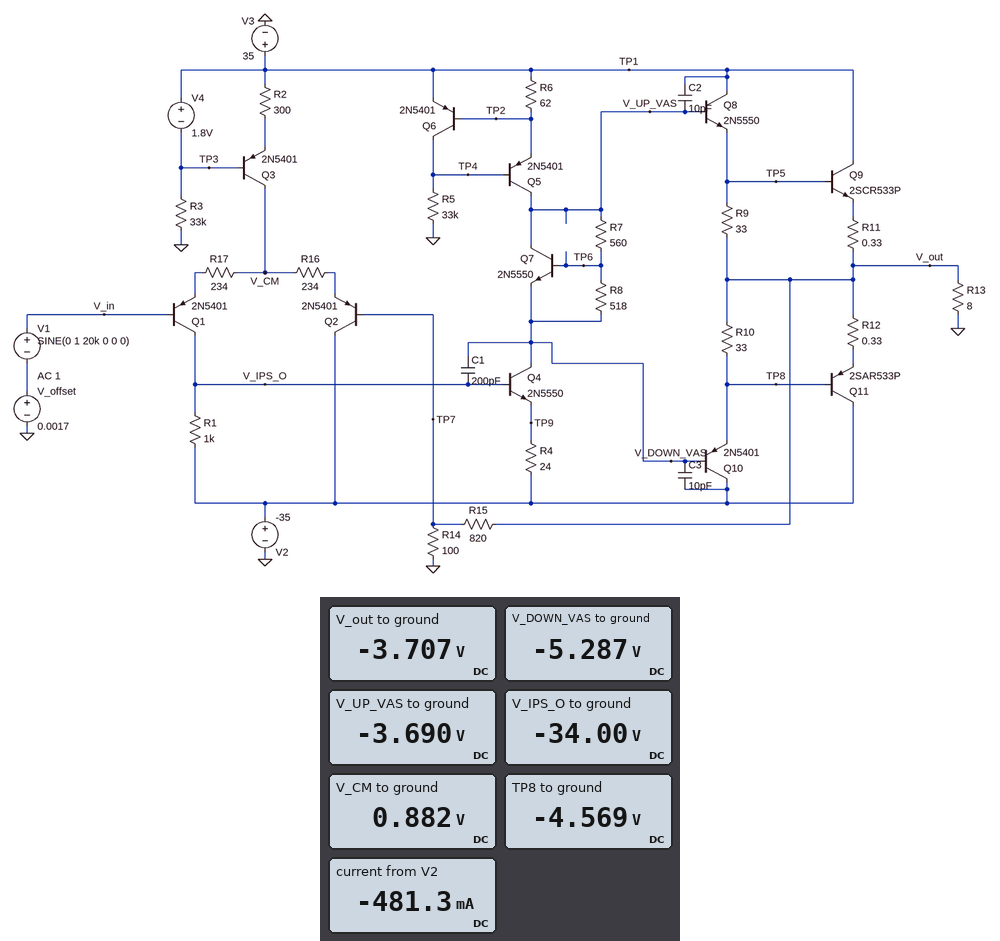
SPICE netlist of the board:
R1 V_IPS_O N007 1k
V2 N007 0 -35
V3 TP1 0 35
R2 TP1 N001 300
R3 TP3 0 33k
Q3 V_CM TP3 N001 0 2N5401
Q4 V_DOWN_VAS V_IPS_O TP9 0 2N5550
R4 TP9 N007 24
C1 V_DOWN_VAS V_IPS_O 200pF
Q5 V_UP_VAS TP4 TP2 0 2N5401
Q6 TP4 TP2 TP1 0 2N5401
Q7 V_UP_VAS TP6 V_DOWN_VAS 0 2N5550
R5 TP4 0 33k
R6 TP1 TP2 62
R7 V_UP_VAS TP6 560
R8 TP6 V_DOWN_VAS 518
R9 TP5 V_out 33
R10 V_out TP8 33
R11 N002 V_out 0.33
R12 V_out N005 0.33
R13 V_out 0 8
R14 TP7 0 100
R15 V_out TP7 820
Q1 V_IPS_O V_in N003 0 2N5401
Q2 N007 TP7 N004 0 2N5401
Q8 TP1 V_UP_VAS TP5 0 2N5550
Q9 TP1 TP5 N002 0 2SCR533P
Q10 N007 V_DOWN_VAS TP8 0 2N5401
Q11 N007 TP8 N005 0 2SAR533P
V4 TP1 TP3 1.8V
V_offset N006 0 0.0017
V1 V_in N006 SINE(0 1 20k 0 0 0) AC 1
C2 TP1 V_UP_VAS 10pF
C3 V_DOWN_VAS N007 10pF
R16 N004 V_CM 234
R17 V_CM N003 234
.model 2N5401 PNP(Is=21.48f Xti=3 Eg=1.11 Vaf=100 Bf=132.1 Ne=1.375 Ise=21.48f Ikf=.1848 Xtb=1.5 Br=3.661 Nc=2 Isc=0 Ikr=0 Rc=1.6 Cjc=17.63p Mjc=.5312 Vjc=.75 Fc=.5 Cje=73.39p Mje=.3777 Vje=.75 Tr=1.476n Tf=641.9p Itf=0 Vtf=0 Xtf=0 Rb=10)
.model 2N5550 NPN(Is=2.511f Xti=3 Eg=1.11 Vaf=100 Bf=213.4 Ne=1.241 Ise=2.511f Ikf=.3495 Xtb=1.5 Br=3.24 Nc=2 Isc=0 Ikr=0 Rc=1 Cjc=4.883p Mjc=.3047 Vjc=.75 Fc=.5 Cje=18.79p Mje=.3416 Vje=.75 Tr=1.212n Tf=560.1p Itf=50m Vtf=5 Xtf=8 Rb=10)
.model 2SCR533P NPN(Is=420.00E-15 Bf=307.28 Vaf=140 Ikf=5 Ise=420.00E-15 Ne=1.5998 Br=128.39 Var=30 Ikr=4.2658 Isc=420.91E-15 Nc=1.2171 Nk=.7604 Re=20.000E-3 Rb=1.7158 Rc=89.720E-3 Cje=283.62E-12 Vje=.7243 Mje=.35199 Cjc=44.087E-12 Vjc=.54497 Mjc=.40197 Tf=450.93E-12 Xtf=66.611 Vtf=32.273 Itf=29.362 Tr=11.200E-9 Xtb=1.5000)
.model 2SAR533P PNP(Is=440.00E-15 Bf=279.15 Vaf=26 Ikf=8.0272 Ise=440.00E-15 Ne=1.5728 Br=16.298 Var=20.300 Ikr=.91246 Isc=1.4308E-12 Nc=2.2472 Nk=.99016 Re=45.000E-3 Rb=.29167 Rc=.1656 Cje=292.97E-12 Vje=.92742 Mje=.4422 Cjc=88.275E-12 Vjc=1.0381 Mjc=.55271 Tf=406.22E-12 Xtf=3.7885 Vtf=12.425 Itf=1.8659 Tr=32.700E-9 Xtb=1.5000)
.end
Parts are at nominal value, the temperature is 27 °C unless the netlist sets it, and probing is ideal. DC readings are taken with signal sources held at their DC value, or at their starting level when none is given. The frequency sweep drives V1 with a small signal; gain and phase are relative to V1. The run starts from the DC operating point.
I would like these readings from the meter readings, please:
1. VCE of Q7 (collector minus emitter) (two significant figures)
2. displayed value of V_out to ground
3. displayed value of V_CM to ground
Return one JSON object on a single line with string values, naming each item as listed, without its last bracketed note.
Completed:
{"VCE of Q7 (collector minus emitter)": "1.6 V", "displayed value of V_out to ground": "-3.707 V", "displayed value of V_CM to ground": "0.882 V"}
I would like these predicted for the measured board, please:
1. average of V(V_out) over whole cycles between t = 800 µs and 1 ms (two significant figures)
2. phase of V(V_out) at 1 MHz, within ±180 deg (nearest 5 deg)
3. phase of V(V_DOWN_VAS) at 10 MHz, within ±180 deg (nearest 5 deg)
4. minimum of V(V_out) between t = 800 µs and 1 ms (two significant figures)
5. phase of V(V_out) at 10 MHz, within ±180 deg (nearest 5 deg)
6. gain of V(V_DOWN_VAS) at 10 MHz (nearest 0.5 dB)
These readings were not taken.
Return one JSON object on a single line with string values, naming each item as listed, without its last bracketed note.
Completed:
{"average of V(V_out) over whole cycles between t = 800 µs and 1 ms": "-3.7 V", "phase of V(V_out) at 1 MHz, within ±180 deg": "-85 deg", "phase of V(V_DOWN_VAS) at 10 MHz, within ±180 deg": "-130 deg", "minimum of V(V_out) between t = 800 µs and 1 ms": "-13 V", "phase of V(V_out) at 10 MHz, within ±180 deg": "-130 deg", "gain of V(V_DOWN_VAS) at 10 MHz": "-16.0 dB"}
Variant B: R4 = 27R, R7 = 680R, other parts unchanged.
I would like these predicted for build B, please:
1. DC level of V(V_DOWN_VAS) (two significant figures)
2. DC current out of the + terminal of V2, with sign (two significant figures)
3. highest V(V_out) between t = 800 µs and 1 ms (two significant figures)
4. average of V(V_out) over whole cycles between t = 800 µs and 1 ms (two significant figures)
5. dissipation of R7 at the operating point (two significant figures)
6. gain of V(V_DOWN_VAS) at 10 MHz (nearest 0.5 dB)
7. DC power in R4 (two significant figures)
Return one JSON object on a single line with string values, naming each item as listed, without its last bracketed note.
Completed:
{"DC level of V(V_DOWN_VAS)": "-5.1 V", "DC current out of the + terminal of V2, with sign": "-460 mA", "highest V(V_out) between t = 800 µs and 1 ms": "5.5 V", "average of V(V_out) over whole cycles between t = 800 µs and 1 ms": "-3.6 V", "dissipation of R7 at the operating point": "1.6 mW", "gain of V(V_DOWN_VAS) at 10 MHz": "-15.5 dB", "DC power in R4": "2.9 mW"}
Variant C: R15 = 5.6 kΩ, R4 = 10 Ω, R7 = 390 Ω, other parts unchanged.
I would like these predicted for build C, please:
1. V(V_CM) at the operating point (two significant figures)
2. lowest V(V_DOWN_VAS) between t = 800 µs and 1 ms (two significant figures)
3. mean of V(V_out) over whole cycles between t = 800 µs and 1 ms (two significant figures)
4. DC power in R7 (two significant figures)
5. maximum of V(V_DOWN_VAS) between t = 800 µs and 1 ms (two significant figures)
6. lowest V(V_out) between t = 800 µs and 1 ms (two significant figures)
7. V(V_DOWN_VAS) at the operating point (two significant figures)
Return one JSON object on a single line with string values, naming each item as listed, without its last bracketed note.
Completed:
{"V(V_CM) at the operating point": "850 mV", "lowest V(V_DOWN_VAS) between t = 800 µs and 1 ms": "-35 V", "mean of V(V_out) over whole cycles between t = 800 µs and 1 ms": "-14 V", "DC power in R7": "900 µW", "maximum of V(V_DOWN_VAS) between t = 800 µs and 1 ms": "18 V", "lowest V(V_out) between t = 800 µs and 1 ms": "-32 V", "V(V_DOWN_VAS) at the operating point": "-29 V"}
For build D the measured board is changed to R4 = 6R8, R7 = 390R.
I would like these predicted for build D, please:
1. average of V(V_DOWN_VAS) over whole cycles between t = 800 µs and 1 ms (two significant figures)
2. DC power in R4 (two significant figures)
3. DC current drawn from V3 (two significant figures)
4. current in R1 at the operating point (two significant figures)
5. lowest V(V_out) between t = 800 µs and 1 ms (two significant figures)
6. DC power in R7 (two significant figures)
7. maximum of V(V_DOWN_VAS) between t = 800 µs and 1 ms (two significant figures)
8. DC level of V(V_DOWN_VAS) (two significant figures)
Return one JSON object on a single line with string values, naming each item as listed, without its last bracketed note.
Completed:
{"average of V(V_DOWN_VAS) over whole cycles between t = 800 µs and 1 ms": "-5.7 V", "DC power in R4": "740 µW", "DC current drawn from V3": "16 mA", "current in R1 at the operating point": "820 µA", "lowest V(V_out) between t = 800 µs and 1 ms": "-14 V", "DC power in R7": "900 µW", "maximum of V(V_DOWN_VAS) between t = 800 µs and 1 ms": "4.9 V", "DC level of V(V_DOWN_VAS)": "-6.2 V"}
